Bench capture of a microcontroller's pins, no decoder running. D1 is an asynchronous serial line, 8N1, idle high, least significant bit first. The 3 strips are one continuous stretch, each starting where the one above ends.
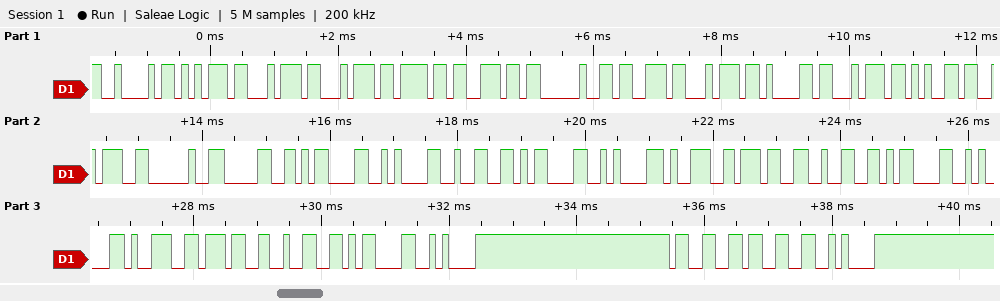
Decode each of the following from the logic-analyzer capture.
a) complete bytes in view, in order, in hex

42 75 74 74 6F 6E 20 73 74 61 74 65 3A 20 30 0D 0A 32 0D 0A 39 37 32 0D 0A 39 37 32 0D 0A 33 33 0A
